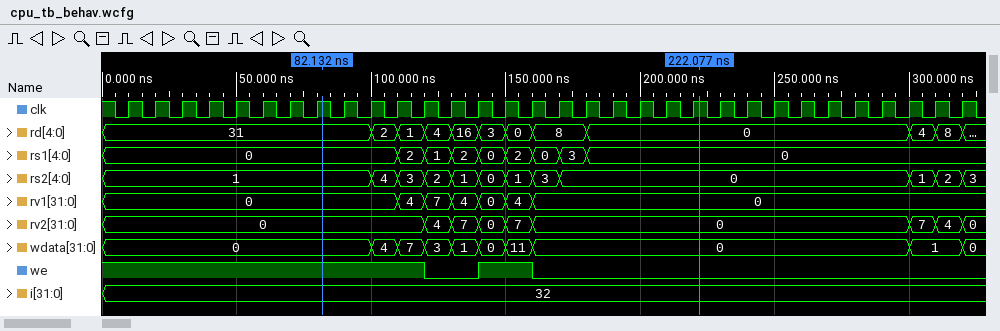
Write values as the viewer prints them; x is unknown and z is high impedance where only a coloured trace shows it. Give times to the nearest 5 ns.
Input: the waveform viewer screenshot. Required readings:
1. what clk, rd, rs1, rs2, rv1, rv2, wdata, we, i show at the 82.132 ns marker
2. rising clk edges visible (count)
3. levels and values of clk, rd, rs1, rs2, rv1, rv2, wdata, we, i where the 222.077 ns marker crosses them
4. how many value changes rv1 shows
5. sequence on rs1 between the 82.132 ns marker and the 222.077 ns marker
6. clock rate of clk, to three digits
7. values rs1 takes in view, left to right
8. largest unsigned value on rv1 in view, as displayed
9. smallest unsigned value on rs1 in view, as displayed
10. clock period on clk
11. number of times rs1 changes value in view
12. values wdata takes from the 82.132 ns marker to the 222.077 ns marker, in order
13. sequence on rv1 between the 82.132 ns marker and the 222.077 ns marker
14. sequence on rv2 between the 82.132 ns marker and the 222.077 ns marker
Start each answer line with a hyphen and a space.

- clk=1, rd=31, rs1=0, rs2=1, rv1=0, rv2=0, wdata=0, we=1, i=32
- 32
- clk=1, rd=0, rs1=0, rs2=0, rv1=0, rv2=0, wdata=0, we=0, i=32
- 6
- 0, 2, 1, 2, 0, 2, 0, 3, 0
- 100 MHz
- 0, 2, 1, 2, 0, 2, 0, 3, 0
- 7
- 0
- 10 ns
- 8
- 0, 4, 7, 3, 1, 0, 11, 0
- 0, 4, 7, 4, 0, 4, 0
- 0, 4, 7, 0, 7, 0
